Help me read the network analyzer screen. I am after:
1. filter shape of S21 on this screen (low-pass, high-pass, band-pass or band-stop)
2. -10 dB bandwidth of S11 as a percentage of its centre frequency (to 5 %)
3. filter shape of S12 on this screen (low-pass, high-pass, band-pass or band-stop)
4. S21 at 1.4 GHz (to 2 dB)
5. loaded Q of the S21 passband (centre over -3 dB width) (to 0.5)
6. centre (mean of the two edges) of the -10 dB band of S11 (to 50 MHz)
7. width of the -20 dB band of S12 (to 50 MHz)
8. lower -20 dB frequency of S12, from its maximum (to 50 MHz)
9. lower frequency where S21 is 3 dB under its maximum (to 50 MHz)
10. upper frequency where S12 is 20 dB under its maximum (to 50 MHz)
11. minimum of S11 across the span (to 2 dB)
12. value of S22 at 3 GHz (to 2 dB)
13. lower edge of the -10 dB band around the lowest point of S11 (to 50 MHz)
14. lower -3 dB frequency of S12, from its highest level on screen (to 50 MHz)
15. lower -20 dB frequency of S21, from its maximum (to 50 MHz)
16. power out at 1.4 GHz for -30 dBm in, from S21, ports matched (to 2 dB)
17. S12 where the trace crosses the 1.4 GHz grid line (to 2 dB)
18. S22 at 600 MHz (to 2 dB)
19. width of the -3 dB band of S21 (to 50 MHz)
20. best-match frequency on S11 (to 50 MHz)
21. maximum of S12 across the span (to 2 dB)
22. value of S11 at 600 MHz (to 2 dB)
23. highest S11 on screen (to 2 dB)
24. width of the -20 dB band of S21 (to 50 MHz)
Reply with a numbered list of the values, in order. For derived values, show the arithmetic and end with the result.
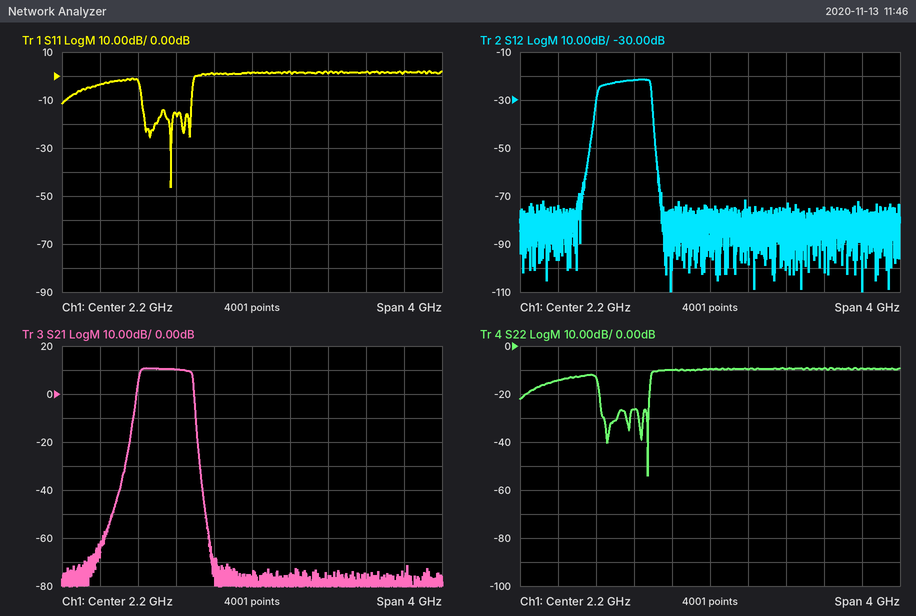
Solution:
1. band-pass
2. 500 MHz / 1.3 GHz ≈ 38.5 %, so 40 % to the nearest 5 %
3. band-pass
4. 10 dB
5. 1.275 GHz / 550 MHz ≈ 2.32, so 2.5 to the nearest 0.5
6. 1.30 GHz
7. 1.60 GHz − 950 MHz = 650 MHz
8. 950 MHz
9. 1.00 GHz
10. 1.60 GHz
11. -46 dB
12. -10 dB
13. 1.05 GHz
14. 1.05 GHz
15. 950 MHz
16. -30 dBm + (10 dB) = -20 dBm
17. -22 dB
18. -14 dB
19. 1.55 GHz − 1.00 GHz = 550 MHz
20. 1.35 GHz
21. -22 dB
22. -4 dB
23. 2 dB
24. 1.60 GHz − 950 MHz = 650 MHz
